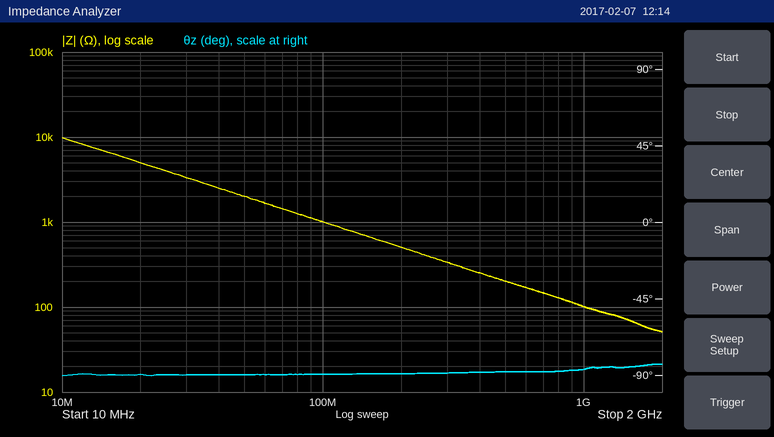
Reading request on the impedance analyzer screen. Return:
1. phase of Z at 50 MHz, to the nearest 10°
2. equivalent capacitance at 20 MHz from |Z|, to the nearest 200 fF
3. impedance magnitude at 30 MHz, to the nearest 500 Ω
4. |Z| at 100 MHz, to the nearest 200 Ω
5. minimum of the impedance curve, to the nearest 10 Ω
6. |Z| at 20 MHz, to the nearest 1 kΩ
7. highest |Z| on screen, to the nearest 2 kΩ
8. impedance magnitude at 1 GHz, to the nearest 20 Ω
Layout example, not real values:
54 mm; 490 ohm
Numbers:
-90°; 1.6 pF; 3.5 kΩ; 1.0 kΩ; 50 Ω; 5 kΩ; 10 kΩ; 100 Ω
